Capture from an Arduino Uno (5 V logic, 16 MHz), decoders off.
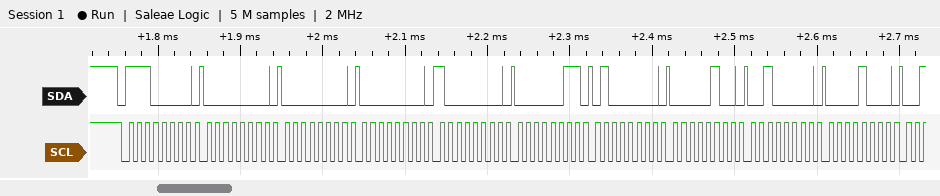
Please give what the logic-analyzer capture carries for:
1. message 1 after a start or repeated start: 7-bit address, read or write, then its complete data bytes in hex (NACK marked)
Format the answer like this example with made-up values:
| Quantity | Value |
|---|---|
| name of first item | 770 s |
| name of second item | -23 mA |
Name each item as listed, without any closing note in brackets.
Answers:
| Quantity | Value |
|---|---|
| message 1 after a start or repeated start: 7-bit address, read or write, then its complete data bytes in hex | 0x70 write: 00 00 00 80 03 40 04 20 08 |
